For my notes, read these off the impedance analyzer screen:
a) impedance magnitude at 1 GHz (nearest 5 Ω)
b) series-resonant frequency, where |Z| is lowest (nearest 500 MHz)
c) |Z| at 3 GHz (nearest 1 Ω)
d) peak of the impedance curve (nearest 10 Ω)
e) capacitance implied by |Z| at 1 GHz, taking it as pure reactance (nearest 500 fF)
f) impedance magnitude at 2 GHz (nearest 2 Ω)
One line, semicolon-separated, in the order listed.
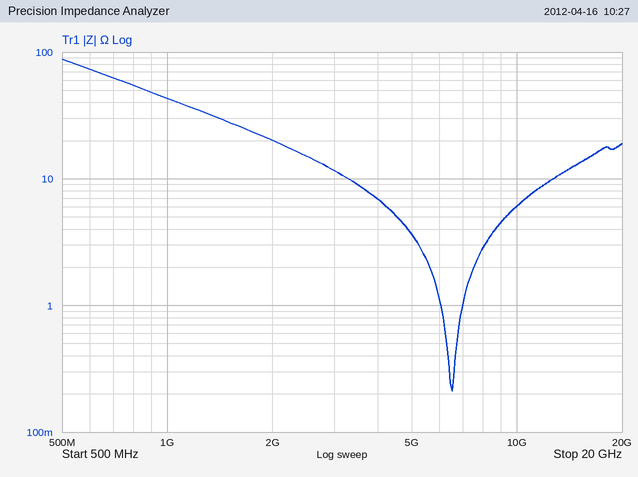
45 Ω; 6.5 GHz; 12 Ω; 90 Ω; 3.5 pF; 20 Ω
